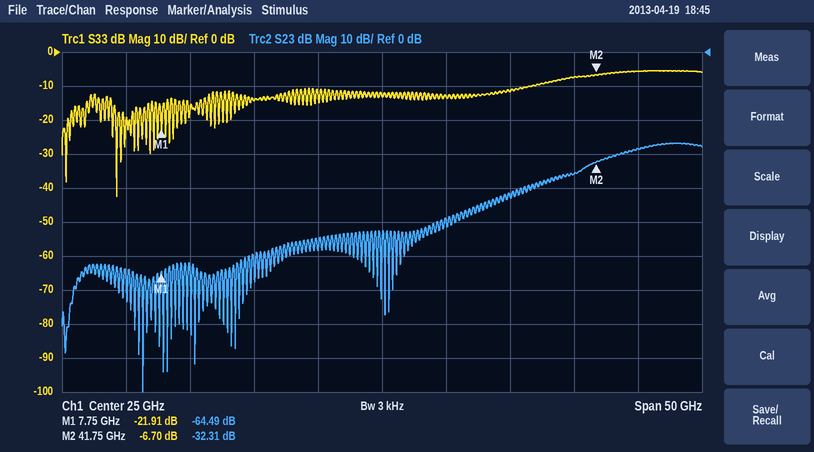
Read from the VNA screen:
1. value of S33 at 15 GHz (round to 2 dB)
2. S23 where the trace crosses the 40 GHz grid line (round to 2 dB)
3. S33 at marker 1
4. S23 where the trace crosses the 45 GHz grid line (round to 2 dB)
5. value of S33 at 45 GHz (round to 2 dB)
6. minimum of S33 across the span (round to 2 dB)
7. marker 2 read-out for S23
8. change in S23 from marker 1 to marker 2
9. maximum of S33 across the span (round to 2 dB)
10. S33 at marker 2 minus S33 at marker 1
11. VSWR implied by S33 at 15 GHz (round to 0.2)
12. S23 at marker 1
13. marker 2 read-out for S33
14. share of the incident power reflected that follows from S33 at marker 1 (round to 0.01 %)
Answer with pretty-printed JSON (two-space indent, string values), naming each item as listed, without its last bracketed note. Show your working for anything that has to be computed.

{
  "value of S33 at 15 GHz": "-14 dB",
  "S23 where the trace crosses the 40 GHz grid line": "-36 dB",
  "S33 at marker 1": "-21.91 dB",
  "S23 where the trace crosses the 45 GHz grid line": "-28 dB",
  "value of S33 at 45 GHz": "-6 dB",
  "minimum of S33 across the span": "-42 dB",
  "marker 2 read-out for S23": "-32.31 dB",
  "change in S23 from marker 1 to marker 2": "-32.31 − (-64.49) = 32.18 dB",
  "maximum of S33 across the span": "-6 dB",
  "S33 at marker 2 minus S33 at marker 1": "-6.7 − (-21.91) = 15.21 dB",
  "VSWR implied by S33 at 15 GHz": "|Γ| = 10^(-14/20) = 0.1995; VSWR = (1 + 0.1995)/(1 − 0.1995) ≈ 1.50, so 1.4 to the nearest 0.2",
  "S23 at marker 1": "-64.49 dB",
  "marker 2 read-out for S33": "-6.70 dB",
  "share of the incident power reflected that follows from S33 at marker 1": "10^(-21.91/10) ≈ 0.64 %"
}
